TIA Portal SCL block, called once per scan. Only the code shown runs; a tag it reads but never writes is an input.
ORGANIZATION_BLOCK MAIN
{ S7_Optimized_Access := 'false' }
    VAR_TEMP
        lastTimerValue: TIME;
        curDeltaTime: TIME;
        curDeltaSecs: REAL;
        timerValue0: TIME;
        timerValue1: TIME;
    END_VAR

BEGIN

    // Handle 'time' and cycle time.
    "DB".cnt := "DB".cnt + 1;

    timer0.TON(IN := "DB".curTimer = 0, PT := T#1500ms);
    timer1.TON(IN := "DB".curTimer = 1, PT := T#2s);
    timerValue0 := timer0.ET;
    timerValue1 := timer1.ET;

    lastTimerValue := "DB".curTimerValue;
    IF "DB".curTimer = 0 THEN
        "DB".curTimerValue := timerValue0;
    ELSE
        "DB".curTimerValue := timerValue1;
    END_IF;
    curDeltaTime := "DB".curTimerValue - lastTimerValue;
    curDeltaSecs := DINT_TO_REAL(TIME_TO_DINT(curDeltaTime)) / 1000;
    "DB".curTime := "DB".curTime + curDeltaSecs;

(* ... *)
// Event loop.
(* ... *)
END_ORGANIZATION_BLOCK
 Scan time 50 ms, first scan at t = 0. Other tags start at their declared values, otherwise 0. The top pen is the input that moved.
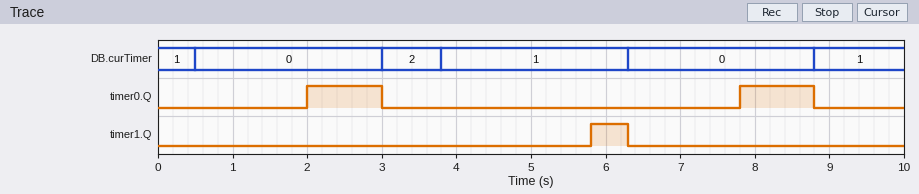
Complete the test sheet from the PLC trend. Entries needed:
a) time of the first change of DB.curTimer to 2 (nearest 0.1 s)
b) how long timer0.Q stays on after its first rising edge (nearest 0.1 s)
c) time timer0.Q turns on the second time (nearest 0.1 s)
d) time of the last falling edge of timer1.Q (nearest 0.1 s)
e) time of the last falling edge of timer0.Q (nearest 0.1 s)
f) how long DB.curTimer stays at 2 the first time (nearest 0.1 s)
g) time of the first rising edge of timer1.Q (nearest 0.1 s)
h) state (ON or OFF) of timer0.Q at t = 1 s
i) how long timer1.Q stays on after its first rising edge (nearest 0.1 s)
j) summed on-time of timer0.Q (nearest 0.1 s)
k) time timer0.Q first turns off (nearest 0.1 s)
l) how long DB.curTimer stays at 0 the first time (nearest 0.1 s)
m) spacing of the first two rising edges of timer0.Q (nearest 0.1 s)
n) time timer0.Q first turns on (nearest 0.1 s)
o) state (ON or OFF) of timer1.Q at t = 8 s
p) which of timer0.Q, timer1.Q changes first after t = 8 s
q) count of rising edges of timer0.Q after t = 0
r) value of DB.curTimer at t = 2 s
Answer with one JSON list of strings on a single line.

["3.0 s", "1.0 s", "7.8 s", "6.3 s", "8.8 s", "0.8 s", "5.8 s", "OFF", "0.5 s", "2.0 s", "3.0 s", "2.5 s", "5.8 s", "2.0 s", "OFF", "timer0.Q", "2", "0"]
